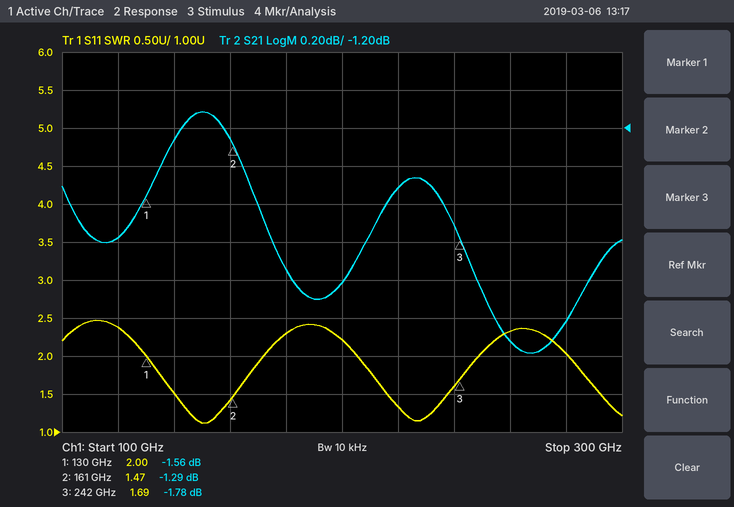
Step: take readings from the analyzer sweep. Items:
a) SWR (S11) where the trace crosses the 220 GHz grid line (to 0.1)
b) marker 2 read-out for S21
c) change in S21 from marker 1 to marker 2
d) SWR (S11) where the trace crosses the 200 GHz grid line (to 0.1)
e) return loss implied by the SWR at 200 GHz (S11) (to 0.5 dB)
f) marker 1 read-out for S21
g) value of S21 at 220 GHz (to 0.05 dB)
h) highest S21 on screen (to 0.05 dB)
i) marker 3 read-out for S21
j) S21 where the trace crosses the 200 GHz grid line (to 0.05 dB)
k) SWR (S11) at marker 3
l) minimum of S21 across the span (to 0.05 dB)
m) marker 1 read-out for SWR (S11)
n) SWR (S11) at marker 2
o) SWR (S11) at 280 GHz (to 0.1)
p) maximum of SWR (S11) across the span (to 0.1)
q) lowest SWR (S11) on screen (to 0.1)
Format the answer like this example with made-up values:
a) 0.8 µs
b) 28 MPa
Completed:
a) 1.3
b) -1.29 dB
c) 0.27 dB
d) 2.2
e) 8.5 dB
f) -1.56 dB
g) -1.50 dB
h) -1.10 dB
i) -1.78 dB
j) -2.00 dB
k) 1.69
l) -2.40 dB
m) 2.00
n) 1.47
o) 2.0
p) 2.5
q) 1.1
